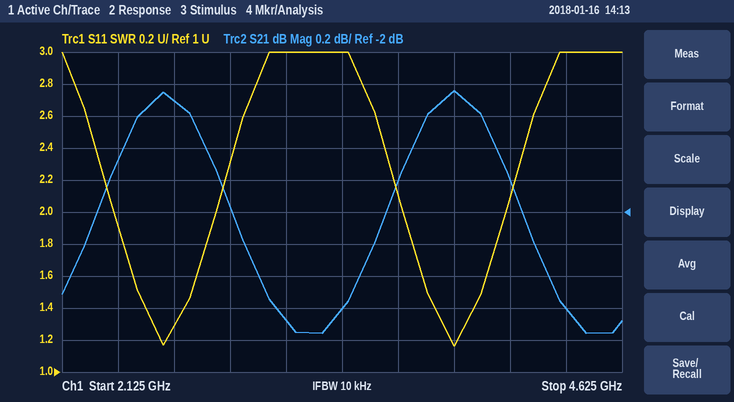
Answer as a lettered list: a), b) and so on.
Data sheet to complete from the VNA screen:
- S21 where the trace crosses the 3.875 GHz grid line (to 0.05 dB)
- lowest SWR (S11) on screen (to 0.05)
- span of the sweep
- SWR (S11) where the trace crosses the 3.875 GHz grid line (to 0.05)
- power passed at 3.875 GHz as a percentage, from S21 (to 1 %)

a) -1.25 dB
b) 1.15
c) 2.5 GHz
d) 1.15
e) 75 %
